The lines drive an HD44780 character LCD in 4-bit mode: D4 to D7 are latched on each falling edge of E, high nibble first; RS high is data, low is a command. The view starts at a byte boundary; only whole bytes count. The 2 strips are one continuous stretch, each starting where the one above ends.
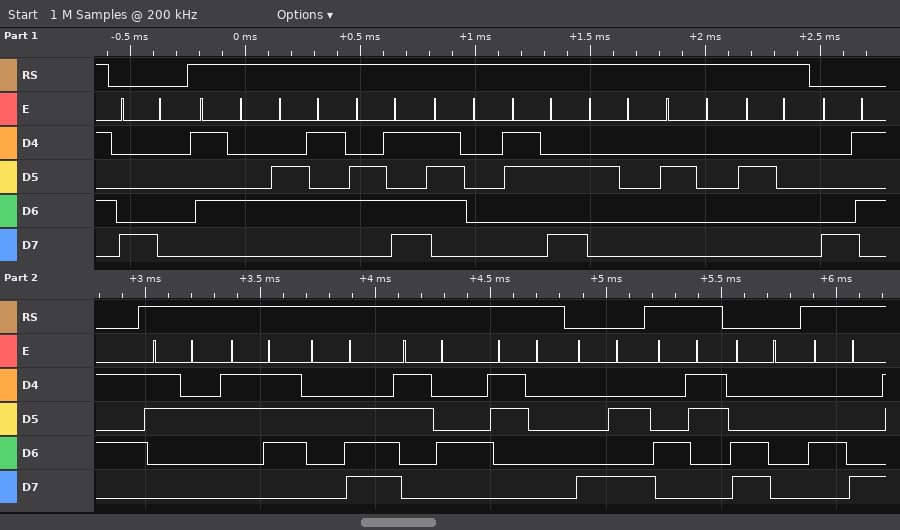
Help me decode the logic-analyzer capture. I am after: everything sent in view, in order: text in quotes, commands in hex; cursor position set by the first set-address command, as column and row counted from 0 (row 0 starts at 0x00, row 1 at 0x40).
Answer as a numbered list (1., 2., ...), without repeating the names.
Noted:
1. 0x80 "Temp:   " 0x85 "27.40" 0x8A "C" 0xC0 "H"
2. column 0, row 0
